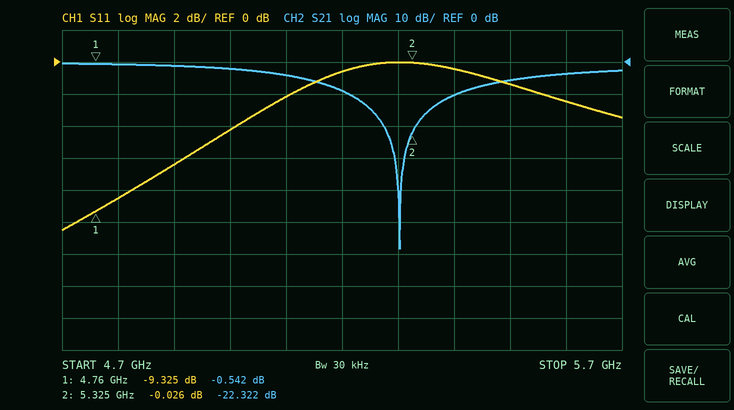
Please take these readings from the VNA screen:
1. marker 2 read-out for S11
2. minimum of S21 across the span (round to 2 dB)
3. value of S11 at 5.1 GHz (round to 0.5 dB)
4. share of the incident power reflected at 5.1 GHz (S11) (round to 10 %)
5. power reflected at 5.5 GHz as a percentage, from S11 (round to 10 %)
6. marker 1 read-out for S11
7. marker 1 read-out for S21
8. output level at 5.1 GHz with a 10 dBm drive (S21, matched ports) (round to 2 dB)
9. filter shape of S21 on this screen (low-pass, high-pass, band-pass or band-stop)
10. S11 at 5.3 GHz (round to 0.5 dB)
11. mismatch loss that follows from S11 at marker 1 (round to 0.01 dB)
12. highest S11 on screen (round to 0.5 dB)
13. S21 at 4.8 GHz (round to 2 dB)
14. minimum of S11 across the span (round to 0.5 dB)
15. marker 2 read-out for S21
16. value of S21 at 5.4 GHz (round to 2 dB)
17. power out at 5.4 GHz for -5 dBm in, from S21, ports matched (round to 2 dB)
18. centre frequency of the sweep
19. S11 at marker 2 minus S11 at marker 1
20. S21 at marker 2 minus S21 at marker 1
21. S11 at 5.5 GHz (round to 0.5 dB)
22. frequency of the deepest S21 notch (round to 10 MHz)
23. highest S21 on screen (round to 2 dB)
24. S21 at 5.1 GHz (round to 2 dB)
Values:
-0.026 dB
-58 dB
-2.0 dB
60 %
70 %
-9.325 dB
-0.542 dB
6 dBm
band-stop
0.0 dB
0.54 dB
0.0 dB
0 dB
-10.5 dB
-22.322 dB
-10 dB
-16 dBm
5.2 GHz
9.299 dB
-21.780 dB
-1.5 dB
5.30 GHz
0 dB
-4 dB
